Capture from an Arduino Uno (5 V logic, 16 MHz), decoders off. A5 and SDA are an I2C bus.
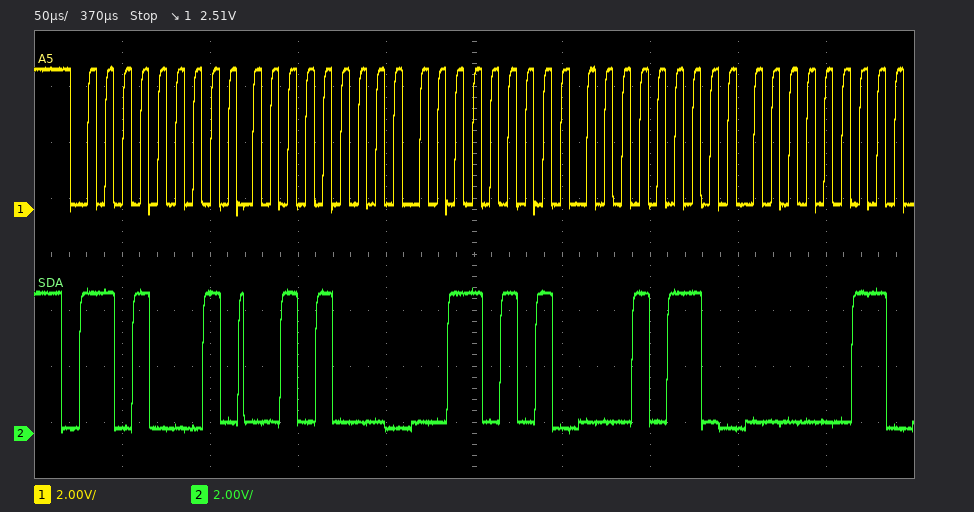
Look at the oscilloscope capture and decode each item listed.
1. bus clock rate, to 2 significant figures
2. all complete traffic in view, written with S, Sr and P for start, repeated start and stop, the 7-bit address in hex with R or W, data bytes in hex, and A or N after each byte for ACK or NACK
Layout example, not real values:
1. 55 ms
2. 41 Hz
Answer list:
1. 100 kHz
2. S 68R A 28 A 35 A 16 A 03 A
